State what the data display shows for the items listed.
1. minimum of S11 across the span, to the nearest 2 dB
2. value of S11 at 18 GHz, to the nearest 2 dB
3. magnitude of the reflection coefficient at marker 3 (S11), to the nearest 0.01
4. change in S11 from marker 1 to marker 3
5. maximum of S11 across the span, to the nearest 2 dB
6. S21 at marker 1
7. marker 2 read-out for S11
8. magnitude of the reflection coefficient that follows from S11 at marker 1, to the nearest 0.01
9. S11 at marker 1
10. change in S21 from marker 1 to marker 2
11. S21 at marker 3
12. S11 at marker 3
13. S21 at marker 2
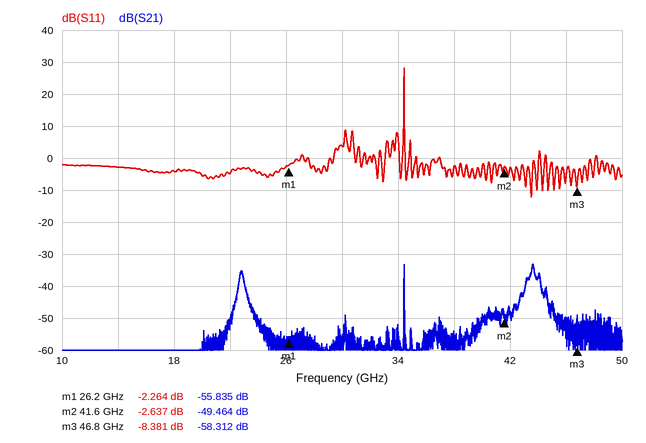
-12 dB
-4 dB
0.38
-6.117 dB
28 dB
-55.835 dB
-2.637 dB
0.77
-2.264 dB
6.371 dB
-58.312 dB
-8.381 dB
-49.464 dB
